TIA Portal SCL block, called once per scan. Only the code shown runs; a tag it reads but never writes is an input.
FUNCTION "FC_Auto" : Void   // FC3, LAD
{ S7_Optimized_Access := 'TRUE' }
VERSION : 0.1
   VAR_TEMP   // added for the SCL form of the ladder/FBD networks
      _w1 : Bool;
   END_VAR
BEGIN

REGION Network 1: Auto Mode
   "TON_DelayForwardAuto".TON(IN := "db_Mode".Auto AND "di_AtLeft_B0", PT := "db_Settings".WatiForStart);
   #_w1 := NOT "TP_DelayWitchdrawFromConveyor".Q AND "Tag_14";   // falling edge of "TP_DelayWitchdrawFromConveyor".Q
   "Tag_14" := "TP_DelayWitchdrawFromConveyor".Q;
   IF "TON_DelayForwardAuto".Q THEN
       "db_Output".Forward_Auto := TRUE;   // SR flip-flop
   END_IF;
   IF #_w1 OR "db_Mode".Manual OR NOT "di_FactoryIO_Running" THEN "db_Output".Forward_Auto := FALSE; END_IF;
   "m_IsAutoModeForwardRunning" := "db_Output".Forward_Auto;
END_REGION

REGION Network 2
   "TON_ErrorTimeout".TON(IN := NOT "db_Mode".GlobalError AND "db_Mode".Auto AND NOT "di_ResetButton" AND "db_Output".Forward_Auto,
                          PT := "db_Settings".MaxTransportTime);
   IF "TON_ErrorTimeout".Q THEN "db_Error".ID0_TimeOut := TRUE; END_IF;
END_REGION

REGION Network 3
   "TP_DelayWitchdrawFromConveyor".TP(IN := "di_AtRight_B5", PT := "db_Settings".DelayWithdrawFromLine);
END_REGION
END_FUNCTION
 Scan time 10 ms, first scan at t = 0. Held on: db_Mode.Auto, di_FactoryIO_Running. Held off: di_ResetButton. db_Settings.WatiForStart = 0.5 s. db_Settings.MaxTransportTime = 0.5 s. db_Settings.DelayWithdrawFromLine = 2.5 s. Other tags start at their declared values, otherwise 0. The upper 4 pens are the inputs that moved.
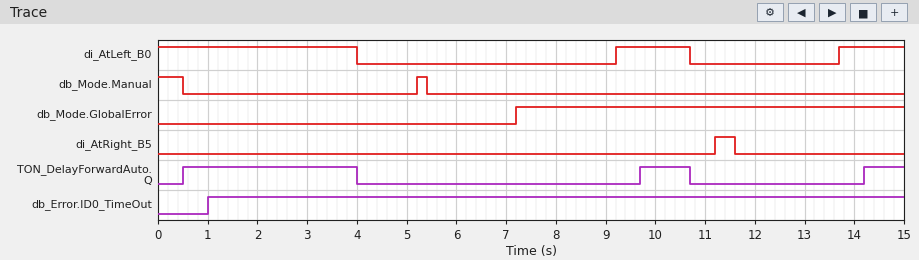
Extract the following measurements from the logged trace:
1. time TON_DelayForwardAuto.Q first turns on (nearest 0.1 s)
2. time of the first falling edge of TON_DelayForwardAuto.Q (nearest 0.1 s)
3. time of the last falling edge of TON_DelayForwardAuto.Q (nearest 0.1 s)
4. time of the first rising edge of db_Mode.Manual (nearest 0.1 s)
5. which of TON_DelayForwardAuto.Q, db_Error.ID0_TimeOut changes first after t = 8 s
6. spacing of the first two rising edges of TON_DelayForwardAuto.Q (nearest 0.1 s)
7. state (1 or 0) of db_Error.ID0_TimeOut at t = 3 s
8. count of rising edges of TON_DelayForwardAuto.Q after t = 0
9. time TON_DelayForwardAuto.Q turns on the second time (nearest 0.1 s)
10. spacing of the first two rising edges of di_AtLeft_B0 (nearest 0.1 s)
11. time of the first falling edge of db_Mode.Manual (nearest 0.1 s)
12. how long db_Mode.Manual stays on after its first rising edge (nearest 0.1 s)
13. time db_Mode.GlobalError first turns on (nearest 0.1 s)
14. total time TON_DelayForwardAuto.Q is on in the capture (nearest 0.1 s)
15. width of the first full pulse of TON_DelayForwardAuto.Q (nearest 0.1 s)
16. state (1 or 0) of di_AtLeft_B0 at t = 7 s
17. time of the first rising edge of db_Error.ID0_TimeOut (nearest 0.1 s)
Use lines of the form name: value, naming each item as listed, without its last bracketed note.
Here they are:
time TON_DelayForwardAuto.Q first turns on: 0.5 s
time of the first falling edge of TON_DelayForwardAuto.Q: 4.0 s
time of the last falling edge of TON_DelayForwardAuto.Q: 10.7 s
time of the first rising edge of db_Mode.Manual: 5.2 s
which of TON_DelayForwardAuto.Q, db_Error.ID0_TimeOut changes first after t = 8 s: TON_DelayForwardAuto.Q
spacing of the first two rising edges of TON_DelayForwardAuto.Q: 9.2 s
state (1 or 0) of db_Error.ID0_TimeOut at t = 3 s: 1
count of rising edges of TON_DelayForwardAuto.Q after t = 0: 3
time TON_DelayForwardAuto.Q turns on the second time: 9.7 s
spacing of the first two rising edges of di_AtLeft_B0: 4.5 s
time of the first falling edge of db_Mode.Manual: 0.5 s
how long db_Mode.Manual stays on after its first rising edge: 0.2 s
time db_Mode.GlobalError first turns on: 7.2 s
total time TON_DelayForwardAuto.Q is on in the capture: 5.3 s
width of the first full pulse of TON_DelayForwardAuto.Q: 3.5 s
state (1 or 0) of di_AtLeft_B0 at t = 7 s: 0
time of the first rising edge of db_Error.ID0_TimeOut: 1.0 s
